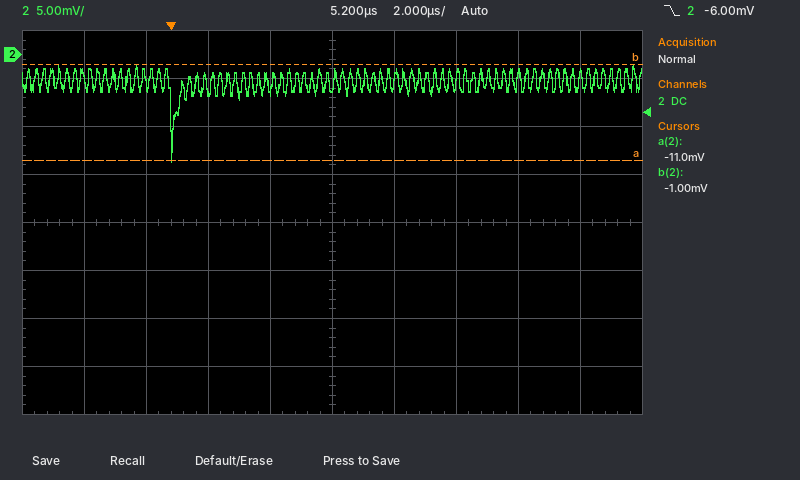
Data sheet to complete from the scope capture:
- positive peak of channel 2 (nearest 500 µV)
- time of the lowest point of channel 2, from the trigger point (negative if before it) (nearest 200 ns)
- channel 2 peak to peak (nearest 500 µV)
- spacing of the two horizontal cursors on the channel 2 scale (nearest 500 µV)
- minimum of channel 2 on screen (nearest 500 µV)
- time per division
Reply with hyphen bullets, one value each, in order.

- -1.0 mV
- 0.0 µs
- 10.0 mV
- 10.0 mV
- -11.0 mV
- 2 µs
